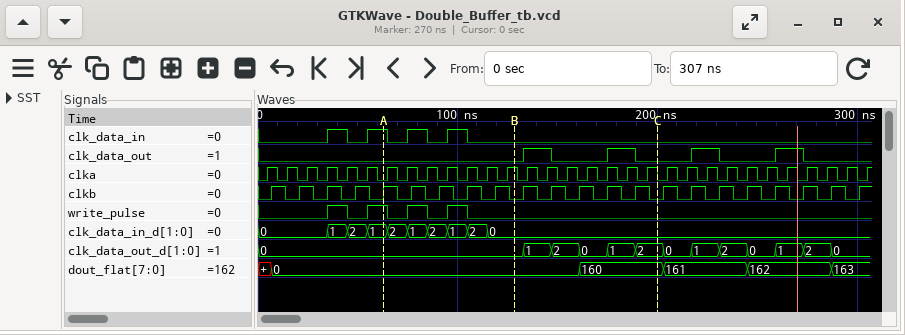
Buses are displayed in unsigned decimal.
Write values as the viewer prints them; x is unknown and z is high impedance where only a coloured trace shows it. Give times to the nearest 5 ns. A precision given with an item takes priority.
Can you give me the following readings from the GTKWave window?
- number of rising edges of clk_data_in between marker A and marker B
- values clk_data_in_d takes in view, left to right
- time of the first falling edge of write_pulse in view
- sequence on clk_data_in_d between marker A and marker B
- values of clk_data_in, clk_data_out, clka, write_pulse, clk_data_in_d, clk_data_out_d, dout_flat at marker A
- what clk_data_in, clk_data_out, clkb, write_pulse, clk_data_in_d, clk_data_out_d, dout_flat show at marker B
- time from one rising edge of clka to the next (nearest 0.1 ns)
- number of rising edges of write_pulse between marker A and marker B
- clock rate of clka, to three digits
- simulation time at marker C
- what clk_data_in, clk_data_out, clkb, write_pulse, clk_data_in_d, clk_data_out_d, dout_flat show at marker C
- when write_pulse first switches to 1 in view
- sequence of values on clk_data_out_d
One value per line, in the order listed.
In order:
2
0, 1, 2, 1, 2, 1, 2, 1, 2, 0
45 ns
1, 2, 1, 2, 1, 2, 0
clk_data_in=1, clk_data_out=0, clka=0, write_pulse=1, clk_data_in_d=1, clk_data_out_d=0, dout_flat=0
clk_data_in=0, clk_data_out=0, clkb=0, write_pulse=0, clk_data_in_d=0, clk_data_out_d=0, dout_flat=0
10 ns
2
100 MHz
200 ns
clk_data_in=0, clk_data_out=0, clkb=0, write_pulse=0, clk_data_in_d=0, clk_data_out_d=2, dout_flat=160
35 ns
0, 1, 2, 0, 1, 2, 0, 1, 2, 0, 1, 2, 0
